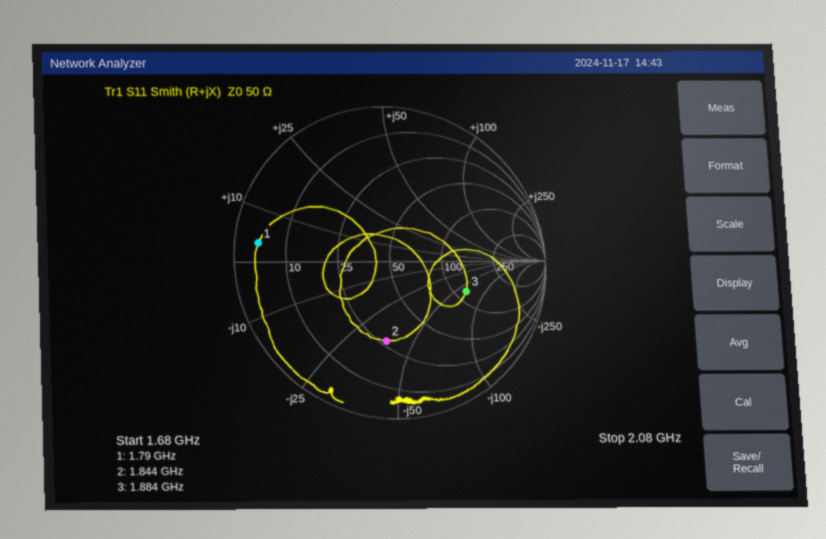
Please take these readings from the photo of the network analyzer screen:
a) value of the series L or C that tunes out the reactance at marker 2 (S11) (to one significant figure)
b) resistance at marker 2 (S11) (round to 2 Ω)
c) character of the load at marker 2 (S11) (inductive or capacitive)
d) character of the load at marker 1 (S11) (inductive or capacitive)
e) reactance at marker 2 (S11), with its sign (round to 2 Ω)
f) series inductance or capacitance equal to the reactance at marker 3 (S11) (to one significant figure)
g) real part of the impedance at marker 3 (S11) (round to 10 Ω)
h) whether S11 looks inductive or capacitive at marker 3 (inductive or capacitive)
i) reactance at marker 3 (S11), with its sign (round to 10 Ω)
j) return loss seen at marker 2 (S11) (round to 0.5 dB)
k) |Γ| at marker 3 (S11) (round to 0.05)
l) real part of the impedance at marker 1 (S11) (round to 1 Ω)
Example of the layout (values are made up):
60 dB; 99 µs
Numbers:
3 nH; 28 Ω; capacitive; inductive; -38 Ω; 1 pF; 120 Ω; capacitive; -60 Ω; 6.0 dB; 0.50; 4 Ω
